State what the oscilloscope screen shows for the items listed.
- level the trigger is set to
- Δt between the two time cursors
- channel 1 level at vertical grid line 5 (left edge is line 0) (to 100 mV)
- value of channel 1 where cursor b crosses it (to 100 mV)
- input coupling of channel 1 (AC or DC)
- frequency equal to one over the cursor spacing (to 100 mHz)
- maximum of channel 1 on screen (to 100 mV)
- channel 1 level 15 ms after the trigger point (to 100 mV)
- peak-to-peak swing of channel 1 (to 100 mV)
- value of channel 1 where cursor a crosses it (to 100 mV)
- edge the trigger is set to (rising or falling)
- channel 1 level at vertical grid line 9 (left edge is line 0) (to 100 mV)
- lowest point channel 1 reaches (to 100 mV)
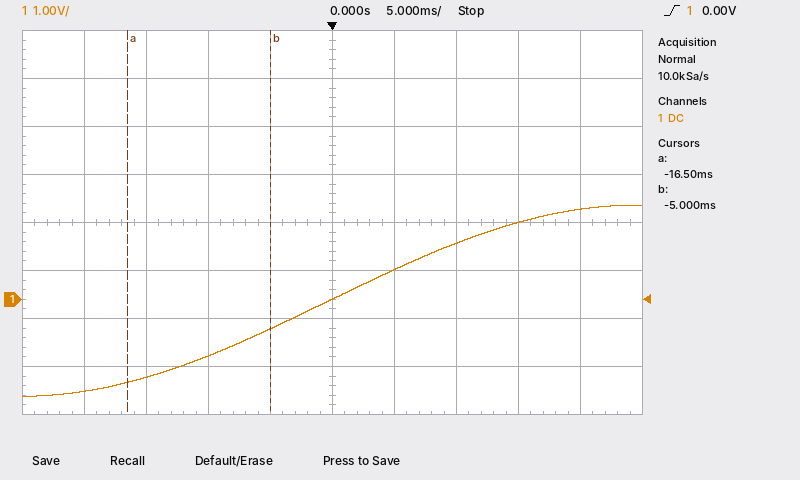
0.00 V
11.5 ms
0.0 V
-600 mV
DC
87.0 Hz
2.0 V
1.6 V
4.0 V
-1.7 V
rising
1.9 V
-2.0 V
